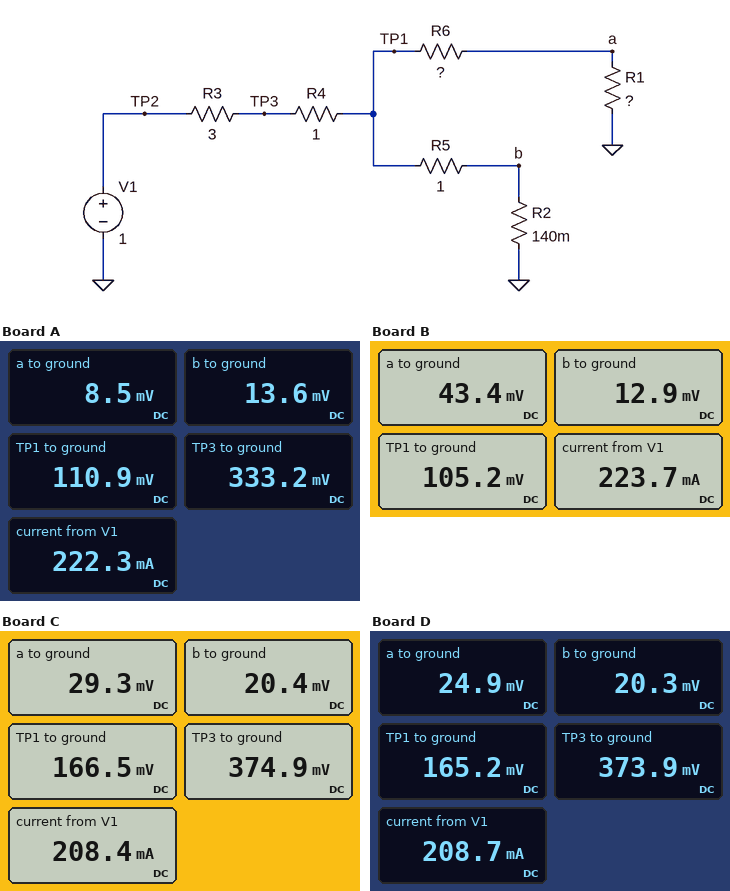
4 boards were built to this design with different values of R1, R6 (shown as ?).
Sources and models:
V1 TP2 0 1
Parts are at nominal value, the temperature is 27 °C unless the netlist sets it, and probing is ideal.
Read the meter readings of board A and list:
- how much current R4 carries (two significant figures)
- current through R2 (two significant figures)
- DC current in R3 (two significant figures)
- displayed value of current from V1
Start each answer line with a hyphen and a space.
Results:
- 220 mA
- 97 mA
- 220 mA
- 222.3 mA
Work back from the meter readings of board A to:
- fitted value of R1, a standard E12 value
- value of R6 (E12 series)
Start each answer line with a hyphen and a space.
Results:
- 0.068 Ω
- 0.82 Ω
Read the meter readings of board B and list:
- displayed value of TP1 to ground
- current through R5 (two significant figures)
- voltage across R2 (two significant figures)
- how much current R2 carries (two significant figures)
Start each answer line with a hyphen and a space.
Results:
- 105.2 mV
- 92 mA
- 13 mV
- 92 mA
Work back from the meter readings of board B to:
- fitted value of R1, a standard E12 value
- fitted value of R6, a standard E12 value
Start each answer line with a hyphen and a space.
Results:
- 0.33 Ω
- 0.47 Ω
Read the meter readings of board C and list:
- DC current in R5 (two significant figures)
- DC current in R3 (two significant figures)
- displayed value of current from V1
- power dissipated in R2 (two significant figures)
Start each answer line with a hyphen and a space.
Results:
- 150 mA
- 210 mA
- 208.4 mA
- 3.0 mW
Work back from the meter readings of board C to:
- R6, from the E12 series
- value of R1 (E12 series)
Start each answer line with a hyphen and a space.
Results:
- 2.2 Ω
- 0.47 Ω
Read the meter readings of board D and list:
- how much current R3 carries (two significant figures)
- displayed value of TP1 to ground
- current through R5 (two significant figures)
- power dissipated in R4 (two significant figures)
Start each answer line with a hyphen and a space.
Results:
- 210 mA
- 165.2 mV
- 140 mA
- 44 mW
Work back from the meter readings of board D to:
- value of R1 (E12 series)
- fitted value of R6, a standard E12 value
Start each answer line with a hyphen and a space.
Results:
- 0.39 Ω
- 2.2 Ω
